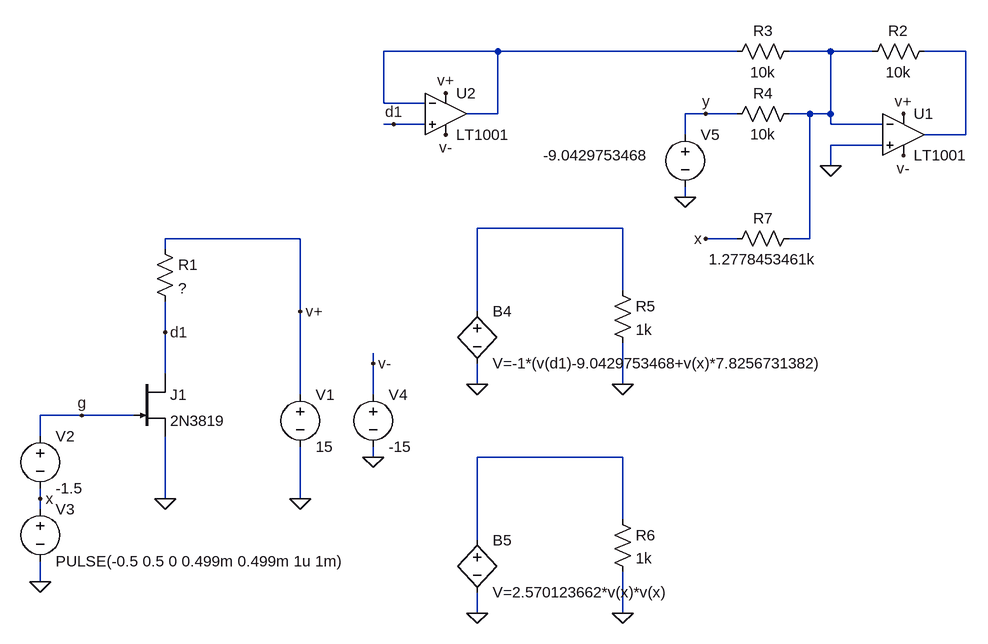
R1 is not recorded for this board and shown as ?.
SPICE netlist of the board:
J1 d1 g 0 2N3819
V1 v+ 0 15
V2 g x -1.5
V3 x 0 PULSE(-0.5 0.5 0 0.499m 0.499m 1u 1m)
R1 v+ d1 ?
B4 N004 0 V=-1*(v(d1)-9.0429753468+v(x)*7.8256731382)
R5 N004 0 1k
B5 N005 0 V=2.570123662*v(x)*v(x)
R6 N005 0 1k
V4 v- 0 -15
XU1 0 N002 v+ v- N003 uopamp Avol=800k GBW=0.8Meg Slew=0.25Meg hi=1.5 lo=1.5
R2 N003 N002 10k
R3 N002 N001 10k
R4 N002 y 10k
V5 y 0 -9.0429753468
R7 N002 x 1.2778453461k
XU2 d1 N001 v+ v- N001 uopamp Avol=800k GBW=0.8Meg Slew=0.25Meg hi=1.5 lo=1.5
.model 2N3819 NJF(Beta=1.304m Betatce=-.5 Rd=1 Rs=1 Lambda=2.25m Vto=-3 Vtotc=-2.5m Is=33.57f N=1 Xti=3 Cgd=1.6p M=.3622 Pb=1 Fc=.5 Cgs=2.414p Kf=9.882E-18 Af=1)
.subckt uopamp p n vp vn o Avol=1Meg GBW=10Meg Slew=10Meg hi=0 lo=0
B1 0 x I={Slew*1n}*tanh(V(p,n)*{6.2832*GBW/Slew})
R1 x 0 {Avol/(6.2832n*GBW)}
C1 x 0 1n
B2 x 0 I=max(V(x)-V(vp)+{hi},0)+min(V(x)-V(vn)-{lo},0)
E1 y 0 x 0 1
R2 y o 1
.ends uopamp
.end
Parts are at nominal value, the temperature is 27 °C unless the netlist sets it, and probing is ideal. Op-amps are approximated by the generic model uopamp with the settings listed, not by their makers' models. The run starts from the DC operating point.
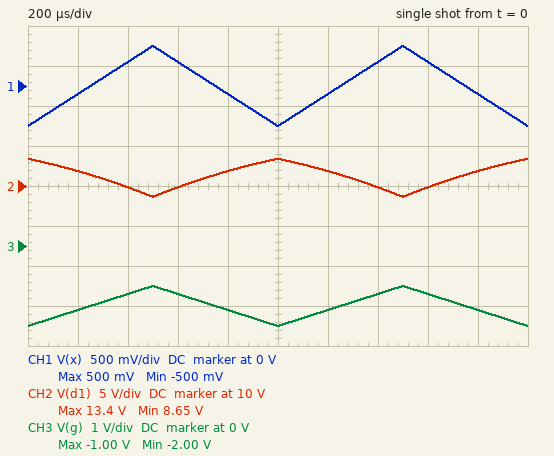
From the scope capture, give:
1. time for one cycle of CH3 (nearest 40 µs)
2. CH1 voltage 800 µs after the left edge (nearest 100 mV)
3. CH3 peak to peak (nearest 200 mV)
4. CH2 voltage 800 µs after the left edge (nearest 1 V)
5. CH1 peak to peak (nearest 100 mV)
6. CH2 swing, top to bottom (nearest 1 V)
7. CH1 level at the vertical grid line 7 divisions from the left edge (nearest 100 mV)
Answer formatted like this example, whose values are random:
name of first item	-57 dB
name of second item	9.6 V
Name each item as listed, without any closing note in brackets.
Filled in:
time for one cycle of CH3	1.00 ms
CH1 voltage 800 µs after the left edge	-100 mV
CH3 peak to peak	1.0 V
CH2 voltage 800 µs after the left edge	12 V
CH1 peak to peak	1.0 V
CH2 swing, top to bottom	5 V
CH1 level at the vertical grid line 7 divisions from the left edge	300 mV
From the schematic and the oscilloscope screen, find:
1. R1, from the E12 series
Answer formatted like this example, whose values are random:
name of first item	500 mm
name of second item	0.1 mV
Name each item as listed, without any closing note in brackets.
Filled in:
R1, from the E12 series	1.2 kΩ
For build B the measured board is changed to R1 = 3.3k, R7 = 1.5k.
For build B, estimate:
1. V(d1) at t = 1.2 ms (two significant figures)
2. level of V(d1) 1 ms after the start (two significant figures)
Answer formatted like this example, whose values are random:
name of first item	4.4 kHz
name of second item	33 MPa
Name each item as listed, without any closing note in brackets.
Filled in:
V(d1) at t = 1.2 ms	6.5 V
level of V(d1) 1 ms after the start	11 V
